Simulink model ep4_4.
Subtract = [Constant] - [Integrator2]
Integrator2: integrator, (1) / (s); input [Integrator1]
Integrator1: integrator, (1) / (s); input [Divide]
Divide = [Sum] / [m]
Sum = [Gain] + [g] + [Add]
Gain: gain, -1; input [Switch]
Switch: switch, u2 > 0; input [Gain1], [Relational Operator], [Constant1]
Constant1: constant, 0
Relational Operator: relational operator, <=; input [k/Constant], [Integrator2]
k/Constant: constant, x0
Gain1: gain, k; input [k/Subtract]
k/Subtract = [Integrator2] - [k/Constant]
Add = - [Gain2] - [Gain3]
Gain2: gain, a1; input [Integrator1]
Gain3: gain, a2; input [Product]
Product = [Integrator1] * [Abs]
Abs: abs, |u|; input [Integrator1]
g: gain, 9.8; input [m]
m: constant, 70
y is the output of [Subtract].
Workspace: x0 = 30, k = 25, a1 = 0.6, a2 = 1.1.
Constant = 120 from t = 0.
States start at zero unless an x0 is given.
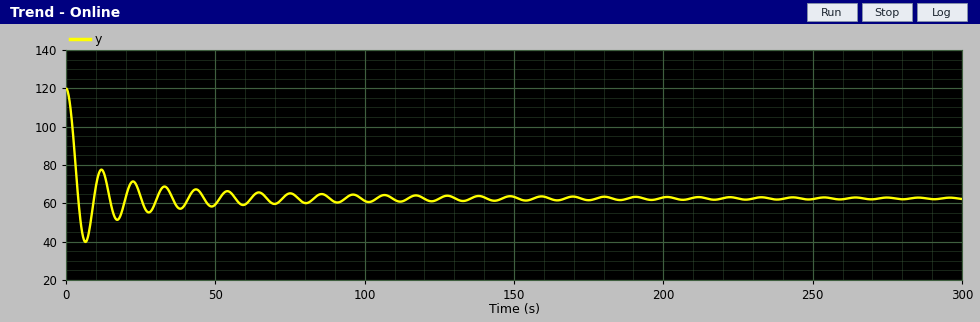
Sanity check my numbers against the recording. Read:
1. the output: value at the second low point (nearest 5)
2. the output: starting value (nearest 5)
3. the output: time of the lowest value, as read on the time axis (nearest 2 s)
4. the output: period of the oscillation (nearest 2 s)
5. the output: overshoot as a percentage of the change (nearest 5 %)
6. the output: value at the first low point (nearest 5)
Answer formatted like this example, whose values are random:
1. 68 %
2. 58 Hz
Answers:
1. 50
2. 120
3. 6 s
4. 10 s
5. 40 %
6. 40
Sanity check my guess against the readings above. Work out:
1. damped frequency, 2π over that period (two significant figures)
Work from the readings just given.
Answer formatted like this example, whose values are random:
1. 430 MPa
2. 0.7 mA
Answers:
1. 0.63 rad/s
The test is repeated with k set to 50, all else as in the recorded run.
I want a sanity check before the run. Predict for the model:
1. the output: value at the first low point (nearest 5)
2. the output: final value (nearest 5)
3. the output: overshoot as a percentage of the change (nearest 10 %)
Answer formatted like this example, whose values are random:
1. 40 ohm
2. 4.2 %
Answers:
1. 60
2. 75
3. 40 %
